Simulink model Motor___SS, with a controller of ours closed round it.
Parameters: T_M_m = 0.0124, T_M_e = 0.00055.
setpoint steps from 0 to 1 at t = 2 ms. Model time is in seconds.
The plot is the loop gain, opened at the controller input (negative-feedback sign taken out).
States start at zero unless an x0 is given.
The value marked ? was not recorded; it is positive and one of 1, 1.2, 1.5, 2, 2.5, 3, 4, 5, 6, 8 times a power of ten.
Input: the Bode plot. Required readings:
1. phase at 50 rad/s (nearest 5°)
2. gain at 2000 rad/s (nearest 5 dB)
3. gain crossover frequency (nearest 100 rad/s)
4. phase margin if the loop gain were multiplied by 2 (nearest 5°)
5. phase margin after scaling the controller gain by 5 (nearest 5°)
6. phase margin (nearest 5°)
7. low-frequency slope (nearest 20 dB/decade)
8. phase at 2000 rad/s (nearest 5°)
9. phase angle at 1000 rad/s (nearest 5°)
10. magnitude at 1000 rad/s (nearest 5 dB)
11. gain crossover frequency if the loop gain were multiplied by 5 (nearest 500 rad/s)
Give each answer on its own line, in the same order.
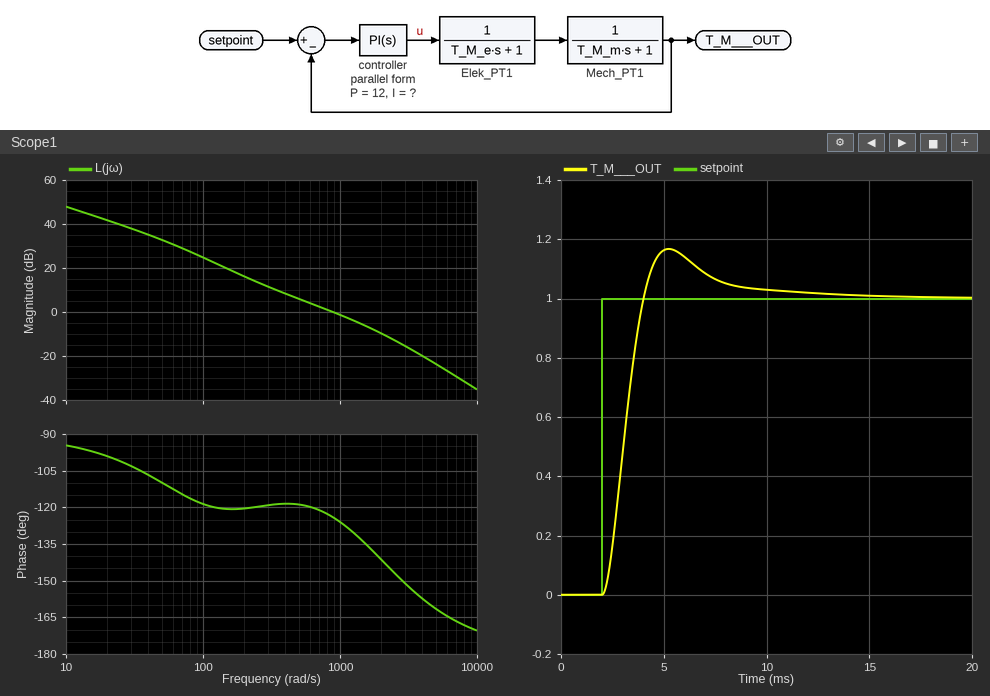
-110°
-10 dB
900 rad/s
45°
30°
55°
-20 dB/decade
-140°
-125°
0 dB
2500 rad/s
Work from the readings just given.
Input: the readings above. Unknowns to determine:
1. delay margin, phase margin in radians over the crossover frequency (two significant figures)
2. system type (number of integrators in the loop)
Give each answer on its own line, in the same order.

0.0011 s
1
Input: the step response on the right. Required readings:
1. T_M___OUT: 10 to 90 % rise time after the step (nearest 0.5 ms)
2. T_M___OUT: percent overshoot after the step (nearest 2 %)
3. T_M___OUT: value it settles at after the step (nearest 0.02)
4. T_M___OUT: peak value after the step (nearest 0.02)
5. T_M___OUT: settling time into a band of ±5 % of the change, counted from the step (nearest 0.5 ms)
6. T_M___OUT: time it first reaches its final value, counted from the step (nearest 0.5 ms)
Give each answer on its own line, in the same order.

1.5 ms
16 %
1.00
1.16
6.0 ms
2.0 ms
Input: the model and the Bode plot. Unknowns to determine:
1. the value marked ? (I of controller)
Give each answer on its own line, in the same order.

2500
